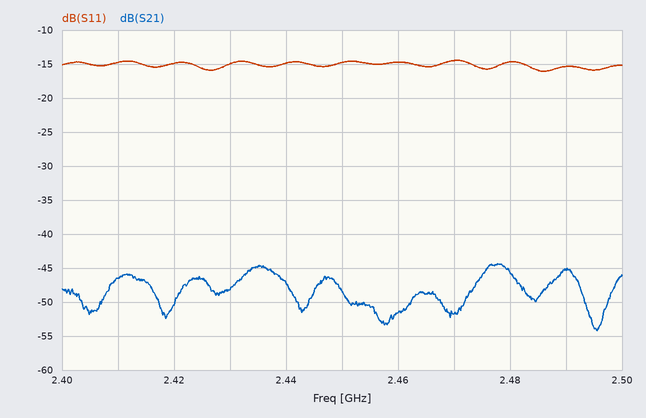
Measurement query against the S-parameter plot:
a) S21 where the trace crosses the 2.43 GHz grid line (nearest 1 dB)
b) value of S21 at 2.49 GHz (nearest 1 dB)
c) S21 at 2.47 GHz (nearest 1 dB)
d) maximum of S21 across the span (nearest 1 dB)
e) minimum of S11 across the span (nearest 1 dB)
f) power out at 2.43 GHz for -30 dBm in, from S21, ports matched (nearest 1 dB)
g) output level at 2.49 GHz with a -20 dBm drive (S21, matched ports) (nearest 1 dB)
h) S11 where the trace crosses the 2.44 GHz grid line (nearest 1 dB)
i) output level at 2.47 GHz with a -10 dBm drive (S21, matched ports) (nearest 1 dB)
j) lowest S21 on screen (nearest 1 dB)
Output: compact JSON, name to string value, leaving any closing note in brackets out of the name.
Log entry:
{"S21 where the trace crosses the 2.43 GHz grid line": "-48 dB", "value of S21 at 2.49 GHz": "-45 dB", "S21 at 2.47 GHz": "-52 dB", "maximum of S21 across the span": "-44 dB", "minimum of S11 across the span": "-16 dB", "power out at 2.43 GHz for -30 dBm in, from S21, ports matched": "-78 dBm", "output level at 2.49 GHz with a -20 dBm drive (S21, matched ports)": "-65 dBm", "S11 where the trace crosses the 2.44 GHz grid line": "-15 dB", "output level at 2.47 GHz with a -10 dBm drive (S21, matched ports)": "-62 dBm", "lowest S21 on screen": "-54 dB"}
